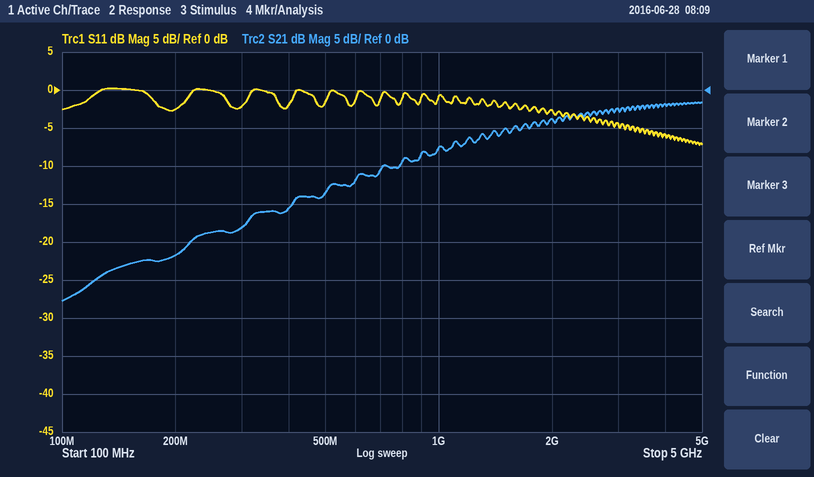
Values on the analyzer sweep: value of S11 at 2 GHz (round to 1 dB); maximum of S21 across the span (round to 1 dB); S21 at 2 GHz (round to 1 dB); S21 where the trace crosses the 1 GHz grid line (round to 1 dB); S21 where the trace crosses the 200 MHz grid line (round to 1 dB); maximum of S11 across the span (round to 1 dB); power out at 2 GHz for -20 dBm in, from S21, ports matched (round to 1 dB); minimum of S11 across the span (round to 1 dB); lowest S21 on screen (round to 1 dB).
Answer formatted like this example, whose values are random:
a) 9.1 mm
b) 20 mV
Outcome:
a) -3 dB
b) -2 dB
c) -4 dB
d) -8 dB
e) -22 dB
f) 0 dB
g) -24 dBm
h) -7 dB
i) -28 dB
